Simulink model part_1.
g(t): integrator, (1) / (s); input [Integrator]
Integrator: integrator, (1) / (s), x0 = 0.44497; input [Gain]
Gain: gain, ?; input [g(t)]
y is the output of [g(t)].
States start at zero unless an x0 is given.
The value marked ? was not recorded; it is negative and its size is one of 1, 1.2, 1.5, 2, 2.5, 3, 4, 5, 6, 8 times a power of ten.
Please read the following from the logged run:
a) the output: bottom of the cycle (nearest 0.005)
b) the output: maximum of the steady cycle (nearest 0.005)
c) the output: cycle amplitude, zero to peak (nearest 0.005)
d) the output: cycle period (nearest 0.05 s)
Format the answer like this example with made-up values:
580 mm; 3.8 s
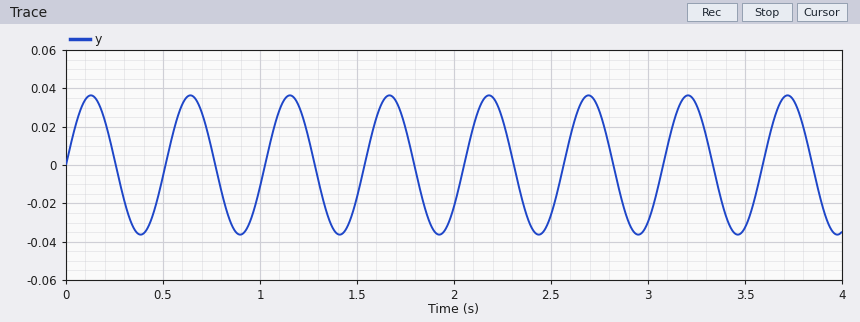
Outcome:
-0.035; 0.035; 0.035; 0.50 s
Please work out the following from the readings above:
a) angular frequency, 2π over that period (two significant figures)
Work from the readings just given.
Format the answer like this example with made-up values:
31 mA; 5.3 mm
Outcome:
13 rad/s
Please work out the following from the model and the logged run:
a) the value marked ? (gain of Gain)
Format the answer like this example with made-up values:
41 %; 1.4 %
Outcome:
-150
